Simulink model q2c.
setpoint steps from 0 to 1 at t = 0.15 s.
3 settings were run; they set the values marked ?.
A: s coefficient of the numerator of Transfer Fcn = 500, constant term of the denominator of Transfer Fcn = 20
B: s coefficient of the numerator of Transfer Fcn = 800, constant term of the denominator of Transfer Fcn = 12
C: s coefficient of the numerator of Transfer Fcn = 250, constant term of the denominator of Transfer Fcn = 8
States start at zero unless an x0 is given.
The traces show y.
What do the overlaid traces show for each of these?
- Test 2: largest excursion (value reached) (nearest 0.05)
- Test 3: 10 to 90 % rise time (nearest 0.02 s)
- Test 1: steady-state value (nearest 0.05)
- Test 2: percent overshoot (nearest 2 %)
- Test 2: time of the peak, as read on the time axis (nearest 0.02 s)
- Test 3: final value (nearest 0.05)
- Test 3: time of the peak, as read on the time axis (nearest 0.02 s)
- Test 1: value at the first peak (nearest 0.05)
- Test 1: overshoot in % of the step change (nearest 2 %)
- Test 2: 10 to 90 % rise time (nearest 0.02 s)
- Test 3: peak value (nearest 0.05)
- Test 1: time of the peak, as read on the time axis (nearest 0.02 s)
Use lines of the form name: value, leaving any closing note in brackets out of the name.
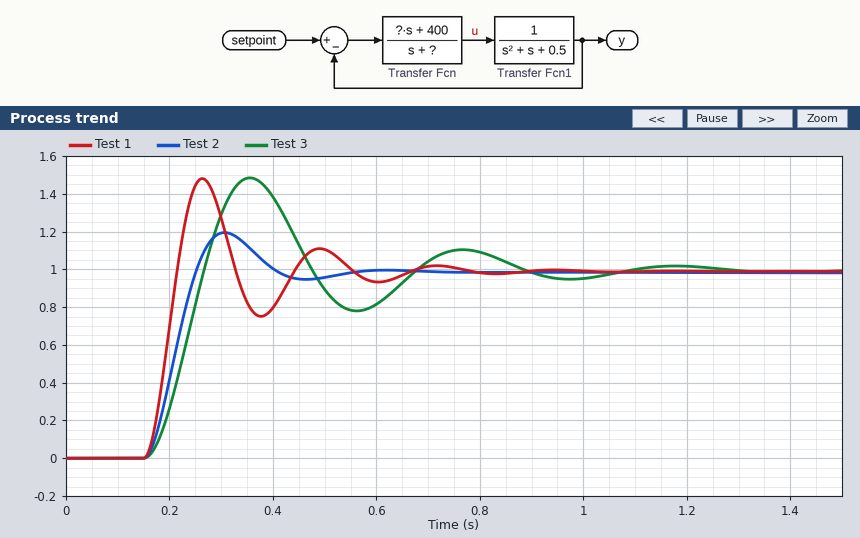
Test 2: largest excursion (value reached): 1.20
Test 3: 10 to 90 % rise time: 0.08 s
Test 1: steady-state value: 1.00
Test 2: percent overshoot: 22 %
Test 2: time of the peak, as read on the time axis: 0.30 s
Test 3: final value: 1.00
Test 3: time of the peak, as read on the time axis: 0.36 s
Test 1: value at the first peak: 1.50
Test 1: overshoot in % of the step change: 50 %
Test 2: 10 to 90 % rise time: 0.06 s
Test 3: peak value: 1.50
Test 1: time of the peak, as read on the time axis: 0.26 s
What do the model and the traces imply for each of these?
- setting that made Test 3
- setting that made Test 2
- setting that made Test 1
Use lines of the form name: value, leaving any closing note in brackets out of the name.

setting that made Test 3: C
setting that made Test 2: A
setting that made Test 1: B
